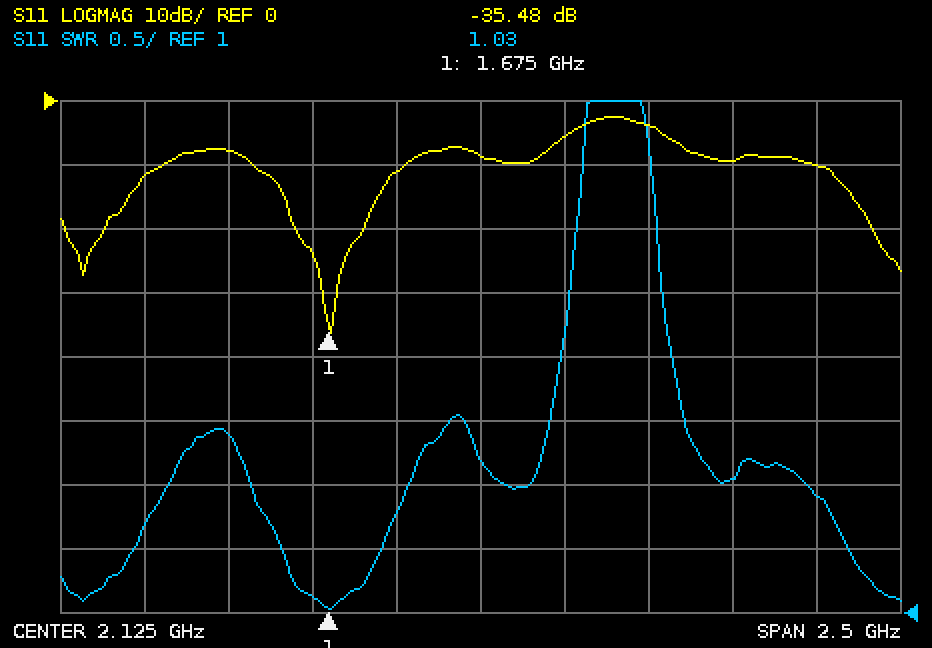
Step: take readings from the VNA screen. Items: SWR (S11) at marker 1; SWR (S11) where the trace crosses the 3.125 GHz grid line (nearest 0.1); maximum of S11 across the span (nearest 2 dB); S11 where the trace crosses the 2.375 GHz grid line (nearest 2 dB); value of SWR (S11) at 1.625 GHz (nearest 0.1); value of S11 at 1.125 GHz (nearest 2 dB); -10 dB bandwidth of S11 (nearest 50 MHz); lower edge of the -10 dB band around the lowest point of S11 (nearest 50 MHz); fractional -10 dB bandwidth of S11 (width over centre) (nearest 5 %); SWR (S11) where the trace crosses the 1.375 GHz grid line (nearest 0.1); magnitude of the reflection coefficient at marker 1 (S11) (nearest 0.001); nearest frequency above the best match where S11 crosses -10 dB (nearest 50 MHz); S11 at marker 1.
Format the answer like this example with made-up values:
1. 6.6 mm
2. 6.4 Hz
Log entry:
1. 1.03
2. 1.9
3. -2 dB
4. -6 dB
5. 1.1
6. -12 dB
7. 450 MHz
8. 1.45 GHz
9. 25 %
10. 2.4
11. 0.017
12. 1.90 GHz
13. -35.48 dB
